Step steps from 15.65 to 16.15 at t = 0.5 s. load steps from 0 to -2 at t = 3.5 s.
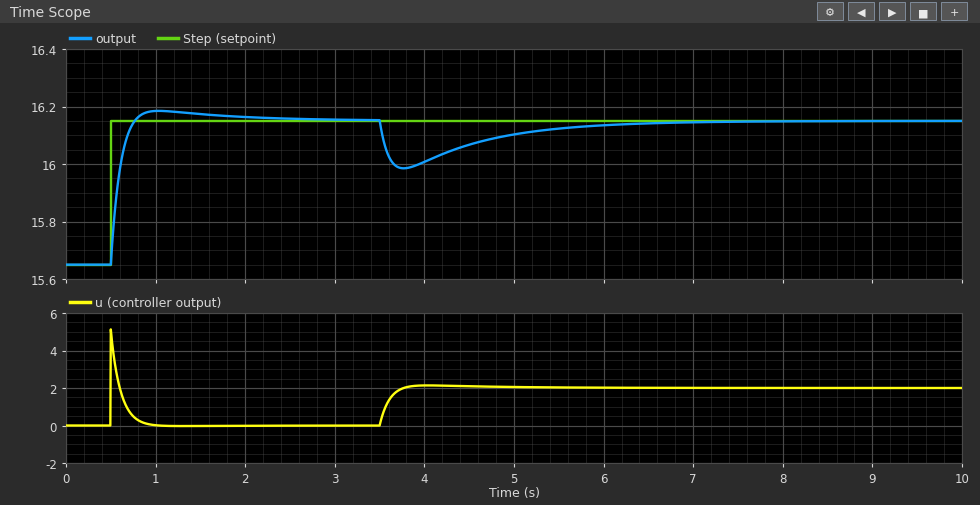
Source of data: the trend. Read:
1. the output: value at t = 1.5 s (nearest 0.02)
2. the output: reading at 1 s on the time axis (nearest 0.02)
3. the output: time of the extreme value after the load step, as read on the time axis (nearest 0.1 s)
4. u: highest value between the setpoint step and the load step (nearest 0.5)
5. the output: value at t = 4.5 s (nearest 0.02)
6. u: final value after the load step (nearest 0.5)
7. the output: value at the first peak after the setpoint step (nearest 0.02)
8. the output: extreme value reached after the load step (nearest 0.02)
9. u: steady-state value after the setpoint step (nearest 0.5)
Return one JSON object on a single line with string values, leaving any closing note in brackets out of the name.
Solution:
{"the output: value at t = 1.5 s": "16.18", "the output: reading at 1 s on the time axis": "16.18", "the output: time of the extreme value after the load step, as read on the time axis": "3.8 s", "u: highest value between the setpoint step and the load step": "5.0", "the output: value at t = 4.5 s": "16.06", "u: final value after the load step": "2.0", "the output: value at the first peak after the setpoint step": "16.18", "the output: extreme value reached after the load step": "15.98", "u: steady-state value after the setpoint step": "0.0"}
